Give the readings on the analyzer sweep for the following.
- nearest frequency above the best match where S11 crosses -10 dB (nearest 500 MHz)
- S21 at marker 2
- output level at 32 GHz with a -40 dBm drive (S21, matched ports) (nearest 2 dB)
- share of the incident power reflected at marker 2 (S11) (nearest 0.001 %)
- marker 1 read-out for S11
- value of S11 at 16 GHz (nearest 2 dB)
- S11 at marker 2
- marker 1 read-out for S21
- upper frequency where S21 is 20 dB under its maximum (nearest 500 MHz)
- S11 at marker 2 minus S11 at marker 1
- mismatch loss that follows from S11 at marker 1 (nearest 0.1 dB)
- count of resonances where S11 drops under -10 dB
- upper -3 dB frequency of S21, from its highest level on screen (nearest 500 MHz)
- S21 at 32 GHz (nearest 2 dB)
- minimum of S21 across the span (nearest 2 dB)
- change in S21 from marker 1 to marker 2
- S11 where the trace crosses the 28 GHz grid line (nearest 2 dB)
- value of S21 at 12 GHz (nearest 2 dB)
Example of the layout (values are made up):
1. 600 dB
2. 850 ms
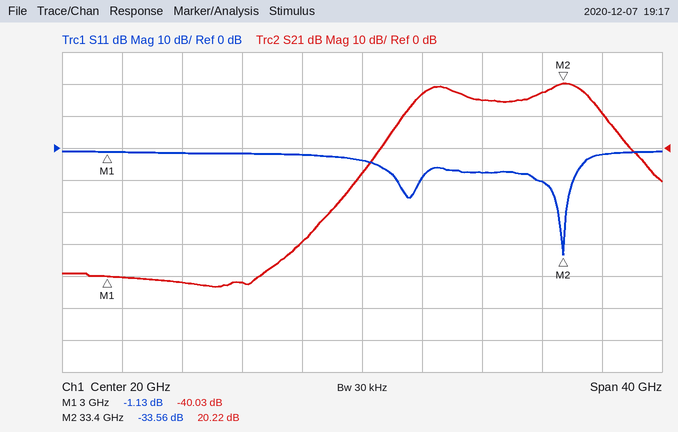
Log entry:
1. 34.0 GHz
2. 20.22 dB
3. -22 dBm
4. 0.044 %
5. -1.13 dB
6. -2 dB
7. -33.56 dB
8. -40.03 dB
9. 38.0 GHz
10. -32.43 dB
11. 6.4 dB
12. 2
13. 35.0 GHz
14. 18 dB
15. -44 dB
16. 60.25 dB
17. -8 dB
18. -42 dB
